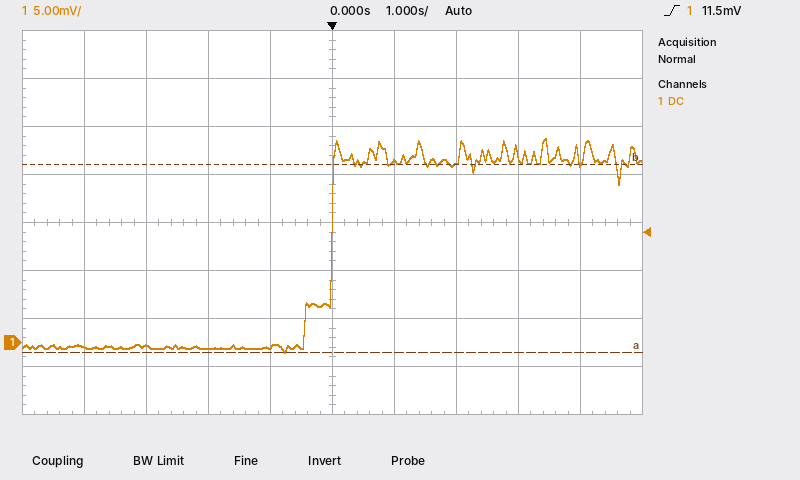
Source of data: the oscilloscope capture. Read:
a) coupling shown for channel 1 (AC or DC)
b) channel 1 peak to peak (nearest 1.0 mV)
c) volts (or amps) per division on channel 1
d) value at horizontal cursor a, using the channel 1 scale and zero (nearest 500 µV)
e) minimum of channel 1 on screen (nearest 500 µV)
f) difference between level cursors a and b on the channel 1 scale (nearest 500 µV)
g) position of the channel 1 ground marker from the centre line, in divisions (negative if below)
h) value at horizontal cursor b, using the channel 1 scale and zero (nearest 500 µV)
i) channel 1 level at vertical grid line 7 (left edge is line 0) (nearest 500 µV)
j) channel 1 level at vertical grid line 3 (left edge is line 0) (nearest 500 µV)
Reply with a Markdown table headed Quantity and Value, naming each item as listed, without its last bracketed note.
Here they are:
| Quantity | Value |
|---|---|
| coupling shown for channel 1 | DC |
| channel 1 peak to peak | 22.0 mV |
| volts (or amps) per division on channel 1 | 5 mV |
| value at horizontal cursor a, using the channel 1 scale and zero | -1.0 mV |
| minimum of channel 1 on screen | -1.0 mV |
| difference between level cursors a and b on the channel 1 scale | 19.5 mV |
| position of the channel 1 ground marker from the centre line, in divisions | -2.5 div |
| value at horizontal cursor b, using the channel 1 scale and zero | 18.5 mV |
| channel 1 level at vertical grid line 7 (left edge is line 0) | 19.0 mV |
| channel 1 level at vertical grid line 3 (left edge is line 0) | -500 µV |
